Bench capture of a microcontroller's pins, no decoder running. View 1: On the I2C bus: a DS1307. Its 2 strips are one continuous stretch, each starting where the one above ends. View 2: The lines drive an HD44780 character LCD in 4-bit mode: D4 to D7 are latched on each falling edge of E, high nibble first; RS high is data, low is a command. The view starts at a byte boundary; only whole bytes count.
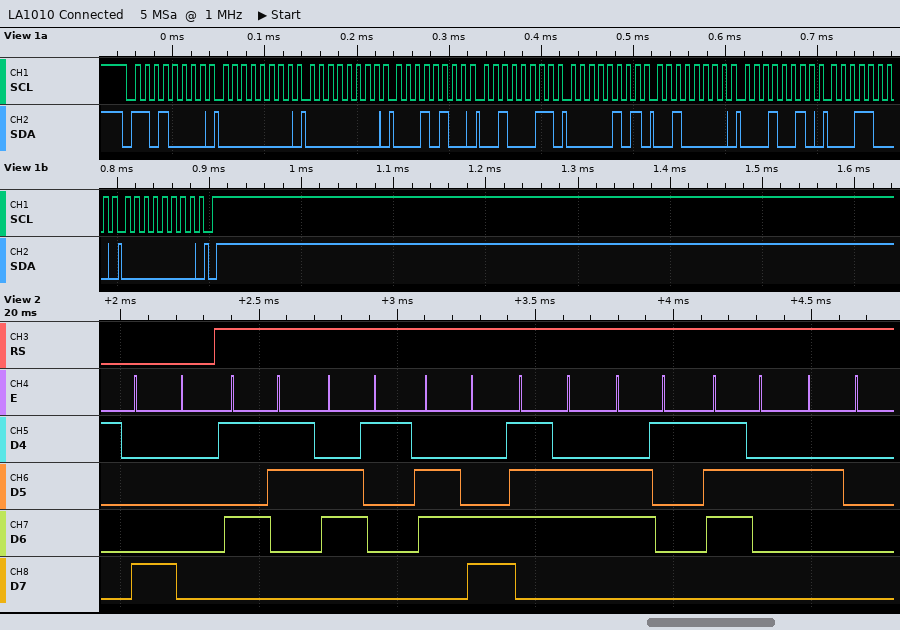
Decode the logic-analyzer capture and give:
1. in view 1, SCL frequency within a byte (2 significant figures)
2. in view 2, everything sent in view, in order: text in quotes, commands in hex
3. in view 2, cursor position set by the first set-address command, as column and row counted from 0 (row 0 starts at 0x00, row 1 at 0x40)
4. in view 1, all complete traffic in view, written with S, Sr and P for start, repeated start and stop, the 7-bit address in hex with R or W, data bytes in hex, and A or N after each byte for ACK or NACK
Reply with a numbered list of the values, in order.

1. 100 kHz
2. 0x80 "Salvar "
3. column 0, row 0
4. S 68W A 00 A 00 A 14 A 23 A 05 A 20 A 12 A 18 A 00 A P
